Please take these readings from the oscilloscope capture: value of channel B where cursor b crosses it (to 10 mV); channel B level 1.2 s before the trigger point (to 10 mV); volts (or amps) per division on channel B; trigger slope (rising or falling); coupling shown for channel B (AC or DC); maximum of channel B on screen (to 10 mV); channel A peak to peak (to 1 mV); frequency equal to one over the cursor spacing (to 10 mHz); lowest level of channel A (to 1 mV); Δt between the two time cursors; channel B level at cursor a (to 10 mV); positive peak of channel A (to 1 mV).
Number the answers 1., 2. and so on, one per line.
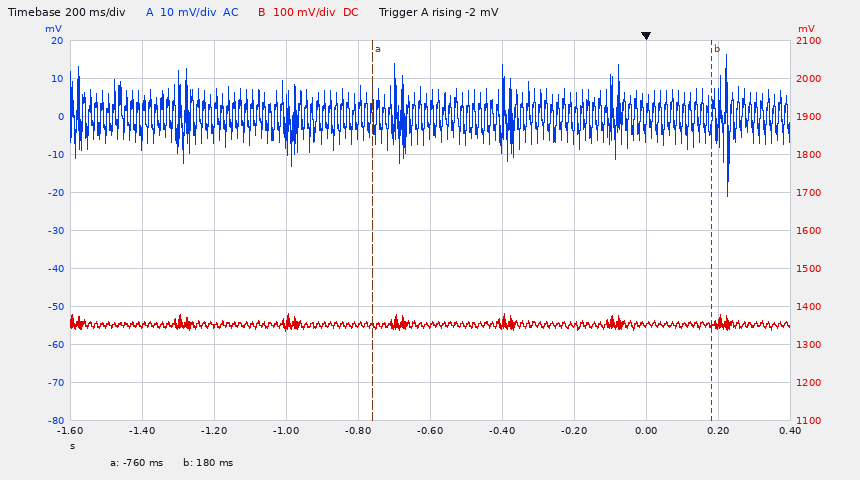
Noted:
1. 1.35 V
2. 1.35 V
3. 100 mV
4. rising
5. DC
6. 1.38 V
7. 37 mV
8. 1.06 Hz
9. -21 mV
10. 940 ms
11. 1.35 V
12. 16 mV
